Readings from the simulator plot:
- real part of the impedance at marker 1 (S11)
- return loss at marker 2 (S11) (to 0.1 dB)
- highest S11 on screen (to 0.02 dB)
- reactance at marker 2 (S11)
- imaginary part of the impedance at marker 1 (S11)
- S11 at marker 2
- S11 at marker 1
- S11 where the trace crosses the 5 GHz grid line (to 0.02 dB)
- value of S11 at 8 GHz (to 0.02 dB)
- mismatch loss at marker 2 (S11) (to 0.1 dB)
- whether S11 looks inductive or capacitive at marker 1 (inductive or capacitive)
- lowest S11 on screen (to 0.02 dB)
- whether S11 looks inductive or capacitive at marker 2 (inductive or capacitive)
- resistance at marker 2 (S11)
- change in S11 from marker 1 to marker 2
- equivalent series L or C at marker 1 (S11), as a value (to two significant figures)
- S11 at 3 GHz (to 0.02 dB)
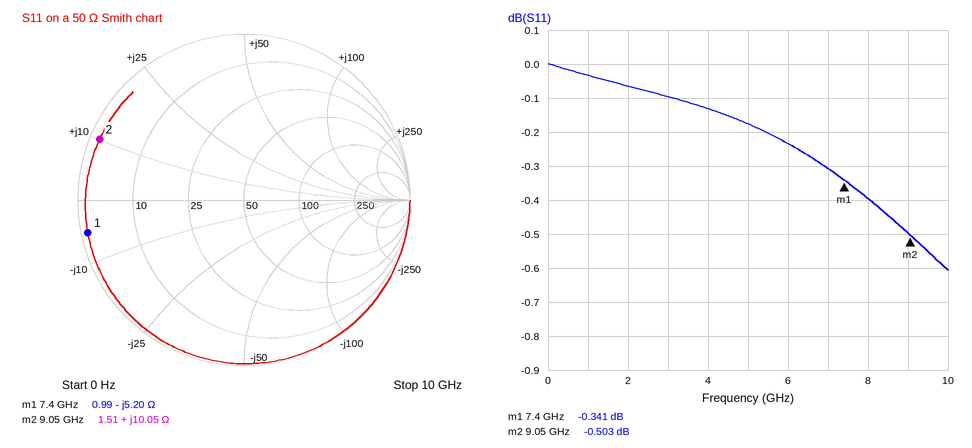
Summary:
0.99 Ω
0.5 dB
0.00 dB
+10.05 Ω
-5.20 Ω
-0.503 dB
-0.341 dB
-0.18 dB
-0.40 dB
9.6 dB
capacitive
-0.60 dB
inductive
1.51 Ω
-0.162 dB
4.1 pF
-0.10 dB
